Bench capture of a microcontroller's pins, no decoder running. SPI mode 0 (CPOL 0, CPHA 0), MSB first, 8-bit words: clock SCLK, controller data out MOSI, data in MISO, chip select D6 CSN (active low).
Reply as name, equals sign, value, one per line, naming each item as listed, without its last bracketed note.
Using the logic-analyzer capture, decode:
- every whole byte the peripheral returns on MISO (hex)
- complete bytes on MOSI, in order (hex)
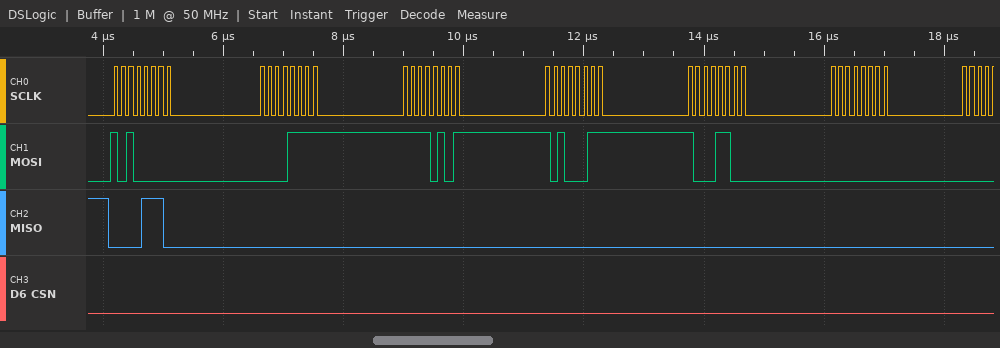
every whole byte the peripheral returns on MISO = 0E 00 00 00 00 00
complete bytes on MOSI, in order = A0 0F F5 A3 8C 00
